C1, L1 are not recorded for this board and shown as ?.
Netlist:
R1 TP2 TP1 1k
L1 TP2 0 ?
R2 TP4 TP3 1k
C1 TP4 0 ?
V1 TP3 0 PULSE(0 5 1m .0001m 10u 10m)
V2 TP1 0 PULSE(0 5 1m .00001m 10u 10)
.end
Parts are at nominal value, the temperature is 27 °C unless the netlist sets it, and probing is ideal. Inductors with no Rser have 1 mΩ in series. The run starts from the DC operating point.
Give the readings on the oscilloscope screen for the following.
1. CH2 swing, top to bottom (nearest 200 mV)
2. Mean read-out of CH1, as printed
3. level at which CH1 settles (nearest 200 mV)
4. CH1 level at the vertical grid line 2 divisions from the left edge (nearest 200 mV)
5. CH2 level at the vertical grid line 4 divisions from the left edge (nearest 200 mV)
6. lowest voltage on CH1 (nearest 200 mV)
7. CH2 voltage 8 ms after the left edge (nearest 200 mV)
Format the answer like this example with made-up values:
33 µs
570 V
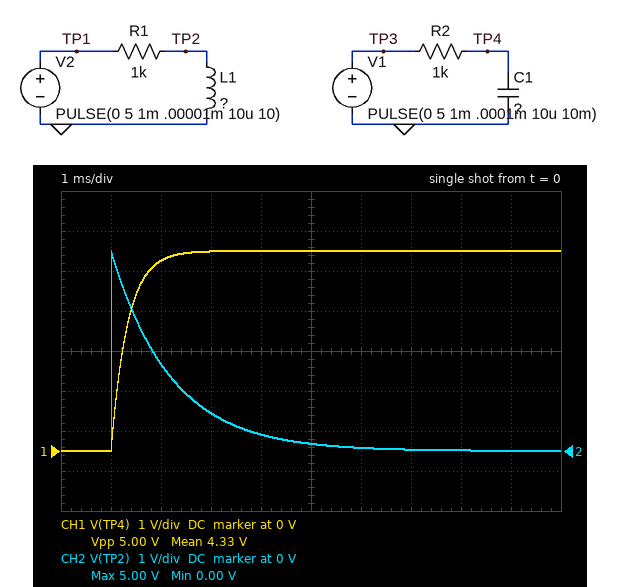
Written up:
5.0 V
4.33 V
5.0 V
4.8 V
400 mV
0 V
0 V
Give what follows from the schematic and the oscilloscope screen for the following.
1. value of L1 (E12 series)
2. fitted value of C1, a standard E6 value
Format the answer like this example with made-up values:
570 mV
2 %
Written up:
1.2 H
330 nF
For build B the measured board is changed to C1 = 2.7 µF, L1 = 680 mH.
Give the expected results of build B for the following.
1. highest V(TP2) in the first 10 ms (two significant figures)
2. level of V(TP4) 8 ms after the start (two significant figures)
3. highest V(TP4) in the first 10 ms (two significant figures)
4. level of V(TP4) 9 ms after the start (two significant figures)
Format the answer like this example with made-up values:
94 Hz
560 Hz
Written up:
5.0 V
4.6 V
4.8 V
4.7 V
